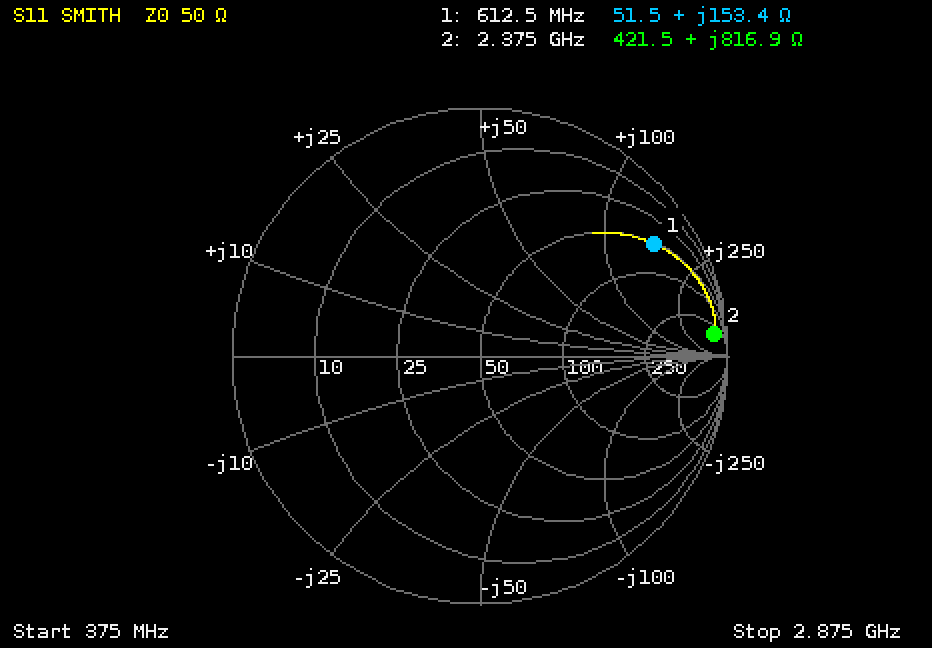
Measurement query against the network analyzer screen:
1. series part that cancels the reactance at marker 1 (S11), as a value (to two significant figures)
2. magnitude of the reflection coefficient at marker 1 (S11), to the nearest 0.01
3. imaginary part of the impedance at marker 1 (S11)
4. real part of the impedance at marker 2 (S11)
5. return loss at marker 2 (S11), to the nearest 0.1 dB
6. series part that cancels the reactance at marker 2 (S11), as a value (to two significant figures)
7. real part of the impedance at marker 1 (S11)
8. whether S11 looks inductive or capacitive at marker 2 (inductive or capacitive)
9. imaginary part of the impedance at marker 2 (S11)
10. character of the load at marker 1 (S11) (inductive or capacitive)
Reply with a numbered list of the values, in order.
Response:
1. 1.7 pF
2. 0.83
3. +153.4 Ω
4. 421.5 Ω
5. 0.4 dB
6. 82 fF
7. 51.5 Ω
8. inductive
9. +816.9 Ω
10. inductive
